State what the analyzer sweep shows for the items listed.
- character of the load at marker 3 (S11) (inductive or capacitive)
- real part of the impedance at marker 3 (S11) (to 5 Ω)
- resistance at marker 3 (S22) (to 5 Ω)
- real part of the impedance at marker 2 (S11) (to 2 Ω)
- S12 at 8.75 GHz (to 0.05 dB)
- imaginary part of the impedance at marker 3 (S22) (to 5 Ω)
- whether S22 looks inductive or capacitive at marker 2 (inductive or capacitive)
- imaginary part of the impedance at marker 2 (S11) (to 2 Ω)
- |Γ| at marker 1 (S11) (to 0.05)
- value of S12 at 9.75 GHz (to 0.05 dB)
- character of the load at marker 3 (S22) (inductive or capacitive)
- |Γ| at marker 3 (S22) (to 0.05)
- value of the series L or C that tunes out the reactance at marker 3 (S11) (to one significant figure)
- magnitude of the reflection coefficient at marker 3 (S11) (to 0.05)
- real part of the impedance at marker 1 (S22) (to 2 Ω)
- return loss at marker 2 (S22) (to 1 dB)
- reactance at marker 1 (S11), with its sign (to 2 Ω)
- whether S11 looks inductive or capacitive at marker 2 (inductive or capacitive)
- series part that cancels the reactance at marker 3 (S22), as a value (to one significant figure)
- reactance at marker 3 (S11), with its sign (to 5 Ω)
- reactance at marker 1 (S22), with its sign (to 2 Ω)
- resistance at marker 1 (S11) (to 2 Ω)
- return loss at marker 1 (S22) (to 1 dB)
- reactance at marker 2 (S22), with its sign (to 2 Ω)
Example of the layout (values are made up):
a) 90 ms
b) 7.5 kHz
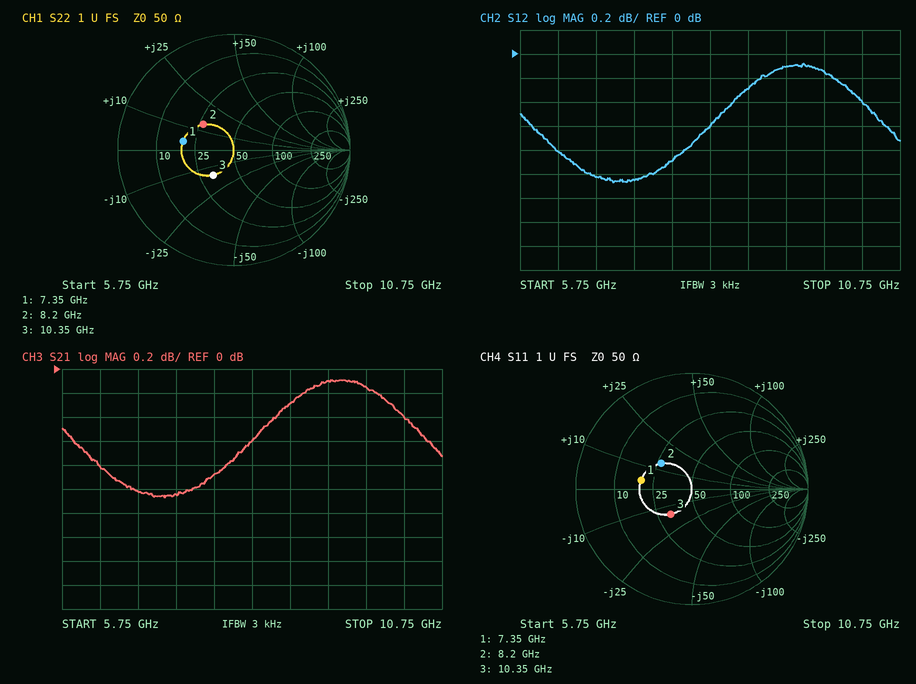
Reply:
a) capacitive
b) 30 Ω
c) 30 Ω
d) 26 Ω
e) -0.30 dB
f) -15 Ω
g) inductive
h) +14 Ω
i) 0.45
j) -0.15 dB
k) capacitive
l) 0.30
m) 200 pH
n) 0.30
o) 20 Ω
p) 9 dB
q) +4 Ω
r) inductive
s) 200 pH
t) -15 Ω
u) +4 Ω
v) 20 Ω
w) 7 dB
x) +14 Ω
